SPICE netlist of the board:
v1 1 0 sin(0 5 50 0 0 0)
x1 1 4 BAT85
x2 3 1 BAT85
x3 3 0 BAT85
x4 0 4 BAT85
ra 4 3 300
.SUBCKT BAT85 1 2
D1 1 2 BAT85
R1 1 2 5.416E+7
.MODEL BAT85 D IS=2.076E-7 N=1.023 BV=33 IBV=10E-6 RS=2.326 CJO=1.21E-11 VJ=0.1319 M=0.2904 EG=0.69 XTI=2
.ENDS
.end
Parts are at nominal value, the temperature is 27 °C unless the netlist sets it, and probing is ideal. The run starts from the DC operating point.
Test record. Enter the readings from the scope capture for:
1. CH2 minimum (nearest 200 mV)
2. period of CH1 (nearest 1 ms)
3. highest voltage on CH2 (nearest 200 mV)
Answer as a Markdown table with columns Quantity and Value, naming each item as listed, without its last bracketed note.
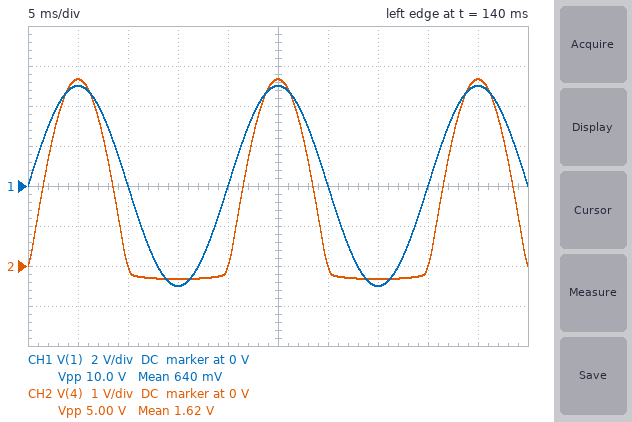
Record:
| Quantity | Value |
|---|---|
| CH2 minimum | -400 mV |
| period of CH1 | 20 ms |
| highest voltage on CH2 | 4.6 V |
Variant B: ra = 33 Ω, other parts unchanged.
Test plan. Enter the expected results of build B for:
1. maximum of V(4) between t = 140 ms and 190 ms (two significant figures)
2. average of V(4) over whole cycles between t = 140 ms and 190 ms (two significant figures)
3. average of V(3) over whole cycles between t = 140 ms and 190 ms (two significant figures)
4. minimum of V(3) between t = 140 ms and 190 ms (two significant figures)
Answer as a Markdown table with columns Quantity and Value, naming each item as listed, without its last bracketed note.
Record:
| Quantity | Value |
|---|---|
| maximum of V(4) between t = 140 ms and 190 ms | 4.4 V |
| average of V(4) over whole cycles between t = 140 ms and 190 ms | 1.1 V |
| average of V(3) over whole cycles between t = 140 ms and 190 ms | -1.1 V |
| minimum of V(3) between t = 140 ms and 190 ms | -4.4 V |
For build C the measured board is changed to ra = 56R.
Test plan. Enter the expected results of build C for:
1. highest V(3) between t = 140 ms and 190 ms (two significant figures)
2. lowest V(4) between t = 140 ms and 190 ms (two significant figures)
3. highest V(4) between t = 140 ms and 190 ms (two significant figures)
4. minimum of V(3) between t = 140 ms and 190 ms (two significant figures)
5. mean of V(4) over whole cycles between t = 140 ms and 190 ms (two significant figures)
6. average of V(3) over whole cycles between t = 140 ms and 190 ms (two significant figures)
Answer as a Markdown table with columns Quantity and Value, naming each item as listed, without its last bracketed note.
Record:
| Quantity | Value |
|---|---|
| highest V(3) between t = 140 ms and 190 ms | 500 mV |
| lowest V(4) between t = 140 ms and 190 ms | -500 mV |
| highest V(4) between t = 140 ms and 190 ms | 4.5 V |
| minimum of V(3) between t = 140 ms and 190 ms | -4.5 V |
| mean of V(4) over whole cycles between t = 140 ms and 190 ms | 1.2 V |
| average of V(3) over whole cycles between t = 140 ms and 190 ms | -1.2 V |
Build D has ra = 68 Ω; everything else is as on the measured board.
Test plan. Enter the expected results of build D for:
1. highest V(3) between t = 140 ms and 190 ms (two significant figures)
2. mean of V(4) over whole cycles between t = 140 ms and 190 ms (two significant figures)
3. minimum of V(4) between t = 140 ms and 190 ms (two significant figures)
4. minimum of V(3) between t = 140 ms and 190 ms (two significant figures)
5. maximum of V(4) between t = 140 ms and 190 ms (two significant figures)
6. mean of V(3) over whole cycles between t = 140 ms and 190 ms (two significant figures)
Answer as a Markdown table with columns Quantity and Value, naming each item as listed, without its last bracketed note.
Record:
| Quantity | Value |
|---|---|
| highest V(3) between t = 140 ms and 190 ms | 470 mV |
| mean of V(4) over whole cycles between t = 140 ms and 190 ms | 1.2 V |
| minimum of V(4) between t = 140 ms and 190 ms | -470 mV |
| minimum of V(3) between t = 140 ms and 190 ms | -4.5 V |
| maximum of V(4) between t = 140 ms and 190 ms | 4.5 V |
| mean of V(3) over whole cycles between t = 140 ms and 190 ms | -1.2 V |
